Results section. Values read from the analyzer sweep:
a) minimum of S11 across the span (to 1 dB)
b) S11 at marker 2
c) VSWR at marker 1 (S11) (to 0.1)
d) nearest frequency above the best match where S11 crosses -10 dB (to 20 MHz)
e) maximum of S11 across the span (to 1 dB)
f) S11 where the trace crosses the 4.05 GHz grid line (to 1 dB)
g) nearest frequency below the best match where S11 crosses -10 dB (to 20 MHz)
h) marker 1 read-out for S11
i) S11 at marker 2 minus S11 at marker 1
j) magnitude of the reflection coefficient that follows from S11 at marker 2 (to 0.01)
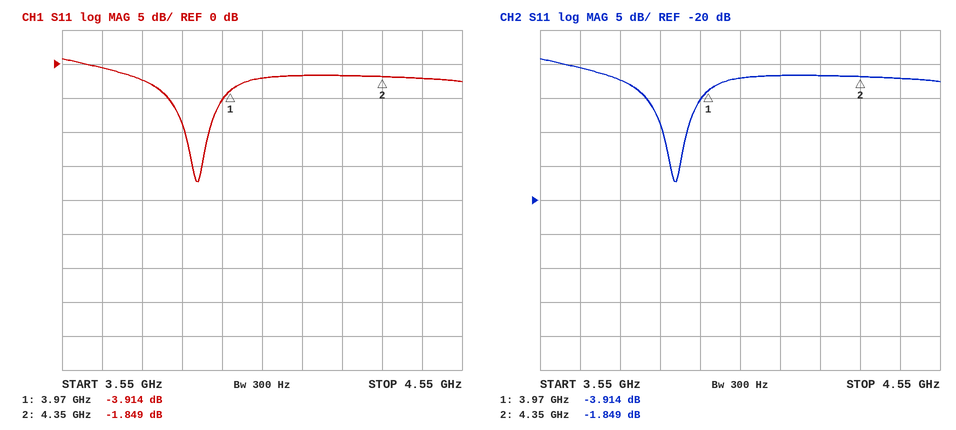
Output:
-17 dB
-1.849 dB
4.5
3.92 GHz
1 dB
-2 dB
3.86 GHz
-3.914 dB
2.065 dB
0.81
